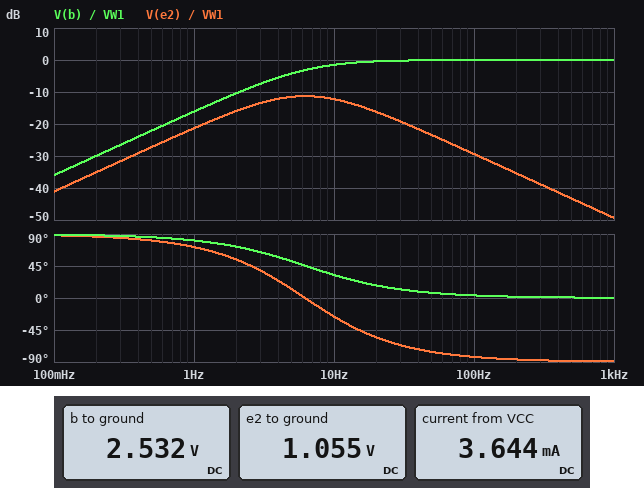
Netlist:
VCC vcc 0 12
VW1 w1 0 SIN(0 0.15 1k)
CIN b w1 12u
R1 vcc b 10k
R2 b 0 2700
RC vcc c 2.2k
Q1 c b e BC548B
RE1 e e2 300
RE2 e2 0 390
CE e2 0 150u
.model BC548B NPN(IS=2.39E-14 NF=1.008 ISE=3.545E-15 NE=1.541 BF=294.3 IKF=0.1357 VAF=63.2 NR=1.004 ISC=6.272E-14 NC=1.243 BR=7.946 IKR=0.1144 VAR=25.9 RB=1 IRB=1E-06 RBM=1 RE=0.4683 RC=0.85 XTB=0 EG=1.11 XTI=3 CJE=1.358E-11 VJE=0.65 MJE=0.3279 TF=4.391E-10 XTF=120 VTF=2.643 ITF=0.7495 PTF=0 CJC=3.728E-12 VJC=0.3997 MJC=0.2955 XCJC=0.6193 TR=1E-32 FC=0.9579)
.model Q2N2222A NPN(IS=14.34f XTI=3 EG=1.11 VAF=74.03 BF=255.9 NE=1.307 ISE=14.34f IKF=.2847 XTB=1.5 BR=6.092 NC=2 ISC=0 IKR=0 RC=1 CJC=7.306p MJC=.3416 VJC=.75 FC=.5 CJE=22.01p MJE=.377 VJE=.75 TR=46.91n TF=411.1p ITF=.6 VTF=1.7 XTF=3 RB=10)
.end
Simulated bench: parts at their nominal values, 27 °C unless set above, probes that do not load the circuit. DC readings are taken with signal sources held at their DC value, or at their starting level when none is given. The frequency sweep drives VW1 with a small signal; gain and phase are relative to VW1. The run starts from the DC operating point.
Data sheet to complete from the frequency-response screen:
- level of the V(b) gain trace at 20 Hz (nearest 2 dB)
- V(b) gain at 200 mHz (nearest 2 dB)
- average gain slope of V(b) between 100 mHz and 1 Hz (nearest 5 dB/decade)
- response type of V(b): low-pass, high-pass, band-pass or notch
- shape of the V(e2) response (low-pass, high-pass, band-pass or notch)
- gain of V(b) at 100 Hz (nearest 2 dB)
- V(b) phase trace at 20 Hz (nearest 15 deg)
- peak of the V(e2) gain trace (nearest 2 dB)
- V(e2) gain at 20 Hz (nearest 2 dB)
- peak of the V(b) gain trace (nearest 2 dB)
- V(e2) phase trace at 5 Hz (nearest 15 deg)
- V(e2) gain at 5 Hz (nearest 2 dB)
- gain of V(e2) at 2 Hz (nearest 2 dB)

0 dB
-30 dB
20 dB/decade
high-pass
band-pass
0 dB
15 deg
-12 dB
-16 dB
0 dB
15 deg
-12 dB
-16 dB
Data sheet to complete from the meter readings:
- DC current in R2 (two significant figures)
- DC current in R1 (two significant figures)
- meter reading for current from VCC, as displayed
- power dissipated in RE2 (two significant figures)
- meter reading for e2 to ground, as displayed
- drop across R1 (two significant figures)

940 µA
950 µA
3.644 mA
2.9 mW
1.055 V
9.5 V
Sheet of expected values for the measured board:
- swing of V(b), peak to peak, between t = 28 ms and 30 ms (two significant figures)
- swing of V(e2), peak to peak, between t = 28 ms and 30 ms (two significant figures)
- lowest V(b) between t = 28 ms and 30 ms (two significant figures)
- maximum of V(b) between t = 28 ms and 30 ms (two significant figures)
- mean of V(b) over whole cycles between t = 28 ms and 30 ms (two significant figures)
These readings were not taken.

300 mV
1.0 mV
2.4 V
2.7 V
2.5 V
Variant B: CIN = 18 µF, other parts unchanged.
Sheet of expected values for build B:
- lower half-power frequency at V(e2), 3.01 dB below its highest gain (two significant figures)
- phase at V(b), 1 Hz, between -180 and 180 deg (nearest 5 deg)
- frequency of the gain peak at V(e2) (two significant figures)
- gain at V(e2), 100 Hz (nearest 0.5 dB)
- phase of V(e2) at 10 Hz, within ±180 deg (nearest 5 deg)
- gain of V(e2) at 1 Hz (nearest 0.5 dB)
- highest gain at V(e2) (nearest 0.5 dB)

2.1 Hz
75 deg
5.1 Hz
-29.5 dB
-35 deg
-18.0 dB
-9.5 dB
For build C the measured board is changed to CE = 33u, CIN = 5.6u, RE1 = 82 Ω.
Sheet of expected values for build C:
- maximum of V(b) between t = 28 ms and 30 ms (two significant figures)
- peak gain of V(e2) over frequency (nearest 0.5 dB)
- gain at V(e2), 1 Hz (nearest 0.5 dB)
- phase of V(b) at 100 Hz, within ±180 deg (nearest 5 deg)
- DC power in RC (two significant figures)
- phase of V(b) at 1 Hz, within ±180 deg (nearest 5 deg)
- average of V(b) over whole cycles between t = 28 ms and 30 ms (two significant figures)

2.5 V
-3.5 dB
-24.5 dB
10 deg
33 mW
85 deg
2.4 V
